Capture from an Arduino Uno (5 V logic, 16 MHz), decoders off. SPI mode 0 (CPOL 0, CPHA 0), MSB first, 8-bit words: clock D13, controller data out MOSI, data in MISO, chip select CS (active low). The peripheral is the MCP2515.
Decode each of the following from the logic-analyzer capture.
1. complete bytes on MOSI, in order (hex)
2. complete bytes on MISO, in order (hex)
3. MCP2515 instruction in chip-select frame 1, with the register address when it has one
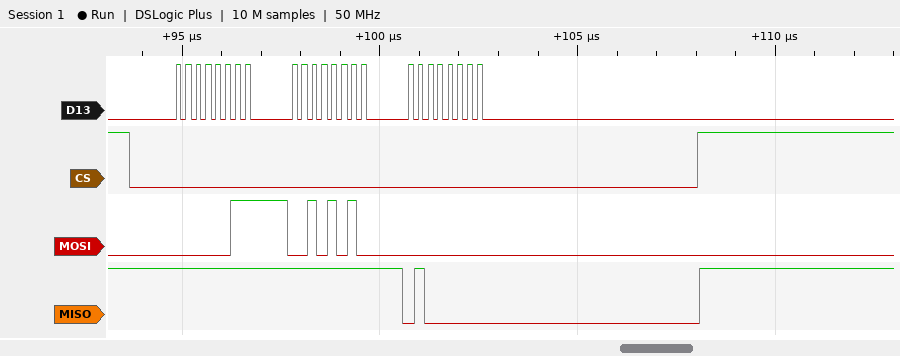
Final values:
0x03 0x2A 0x00
0xFF 0xFF 0x40
READ 0x2A
